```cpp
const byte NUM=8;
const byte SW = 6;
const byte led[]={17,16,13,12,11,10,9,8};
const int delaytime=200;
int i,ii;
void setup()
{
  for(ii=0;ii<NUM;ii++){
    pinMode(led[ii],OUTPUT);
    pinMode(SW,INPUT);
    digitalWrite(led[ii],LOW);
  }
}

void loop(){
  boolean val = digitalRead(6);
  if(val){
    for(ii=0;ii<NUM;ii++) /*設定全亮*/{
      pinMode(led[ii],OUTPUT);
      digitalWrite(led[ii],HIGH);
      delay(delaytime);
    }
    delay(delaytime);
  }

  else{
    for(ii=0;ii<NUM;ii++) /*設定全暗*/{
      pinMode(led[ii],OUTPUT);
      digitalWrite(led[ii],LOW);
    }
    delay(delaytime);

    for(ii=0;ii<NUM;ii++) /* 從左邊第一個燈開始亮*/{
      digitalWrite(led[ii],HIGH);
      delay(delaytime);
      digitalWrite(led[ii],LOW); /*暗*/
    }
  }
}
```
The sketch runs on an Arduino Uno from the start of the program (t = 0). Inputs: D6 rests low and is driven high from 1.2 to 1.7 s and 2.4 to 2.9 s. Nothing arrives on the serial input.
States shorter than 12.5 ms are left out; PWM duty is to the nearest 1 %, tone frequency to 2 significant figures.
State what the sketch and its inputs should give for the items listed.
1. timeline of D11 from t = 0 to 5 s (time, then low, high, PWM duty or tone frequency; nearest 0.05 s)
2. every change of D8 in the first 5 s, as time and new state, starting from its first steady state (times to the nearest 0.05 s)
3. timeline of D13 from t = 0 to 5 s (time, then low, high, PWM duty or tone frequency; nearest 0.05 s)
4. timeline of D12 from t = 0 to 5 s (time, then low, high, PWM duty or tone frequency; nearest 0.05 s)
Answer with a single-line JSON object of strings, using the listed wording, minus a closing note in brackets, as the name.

{"timeline of D11 from t = 0 to 5 s": "0 s low; 1 s high; 1.2 s low; 2.8 s high; 3 s low; 4.6 s high; 4.8 s low", "every change of D8 in the first 5 s, as time and new state, starting from its first steady state": "0 s low; 1.6 s high; 1.8 s low; 3.4 s high; 3.6 s low", "timeline of D13 from t = 0 to 5 s": "0 s low; 0.6 s high; 0.8 s low; 2.4 s high; 2.6 s low; 4.2 s high; 4.4 s low", "timeline of D12 from t = 0 to 5 s": "0 s low; 0.8 s high; 1 s low; 2.6 s high; 2.8 s low; 4.4 s high; 4.6 s low"}
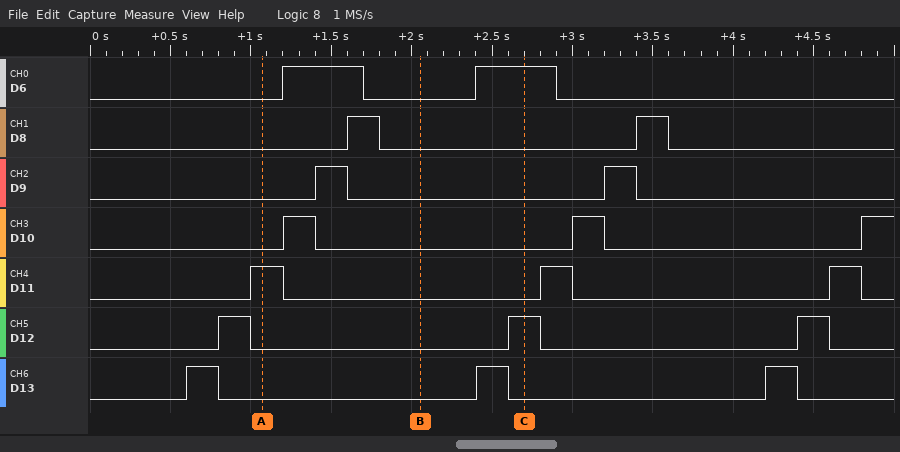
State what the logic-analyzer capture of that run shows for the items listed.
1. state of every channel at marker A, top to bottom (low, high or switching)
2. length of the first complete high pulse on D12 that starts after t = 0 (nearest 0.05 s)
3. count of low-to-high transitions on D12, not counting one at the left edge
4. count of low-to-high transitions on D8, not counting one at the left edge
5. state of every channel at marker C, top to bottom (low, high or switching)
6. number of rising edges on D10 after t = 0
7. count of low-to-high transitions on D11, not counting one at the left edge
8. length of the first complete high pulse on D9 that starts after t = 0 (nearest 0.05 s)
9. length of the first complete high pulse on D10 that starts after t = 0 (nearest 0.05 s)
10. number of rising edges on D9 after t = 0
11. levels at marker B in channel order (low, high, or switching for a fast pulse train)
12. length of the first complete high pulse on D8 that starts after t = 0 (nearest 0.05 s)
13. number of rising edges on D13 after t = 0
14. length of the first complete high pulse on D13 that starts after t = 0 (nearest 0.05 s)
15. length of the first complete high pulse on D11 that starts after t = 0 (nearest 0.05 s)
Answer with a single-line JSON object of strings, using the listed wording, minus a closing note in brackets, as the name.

{"state of every channel at marker A, top to bottom": "D6 low, D8 low, D9 low, D10 low, D11 high, D12 low, D13 low", "length of the first complete high pulse on D12 that starts after t = 0": "0.20 s", "count of low-to-high transitions on D12, not counting one at the left edge": "3", "count of low-to-high transitions on D8, not counting one at the left edge": "2", "state of every channel at marker C, top to bottom": "D6 high, D8 low, D9 low, D10 low, D11 low, D12 high, D13 low", "number of rising edges on D10 after t = 0": "3", "count of low-to-high transitions on D11, not counting one at the left edge": "3", "length of the first complete high pulse on D9 that starts after t = 0": "0.20 s", "length of the first complete high pulse on D10 that starts after t = 0": "0.20 s", "number of rising edges on D9 after t = 0": "2", "levels at marker B in channel order": "D6 low, D8 low, D9 low, D10 low, D11 low, D12 low, D13 low", "length of the first complete high pulse on D8 that starts after t = 0": "0.20 s", "number of rising edges on D13 after t = 0": "3", "length of the first complete high pulse on D13 that starts after t = 0": "0.20 s", "length of the first complete high pulse on D11 that starts after t = 0": "0.20 s"}
